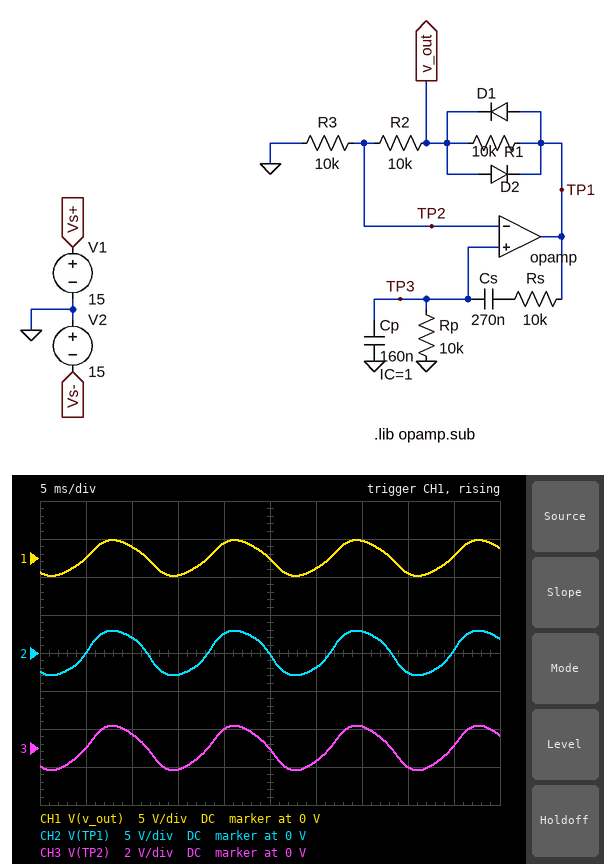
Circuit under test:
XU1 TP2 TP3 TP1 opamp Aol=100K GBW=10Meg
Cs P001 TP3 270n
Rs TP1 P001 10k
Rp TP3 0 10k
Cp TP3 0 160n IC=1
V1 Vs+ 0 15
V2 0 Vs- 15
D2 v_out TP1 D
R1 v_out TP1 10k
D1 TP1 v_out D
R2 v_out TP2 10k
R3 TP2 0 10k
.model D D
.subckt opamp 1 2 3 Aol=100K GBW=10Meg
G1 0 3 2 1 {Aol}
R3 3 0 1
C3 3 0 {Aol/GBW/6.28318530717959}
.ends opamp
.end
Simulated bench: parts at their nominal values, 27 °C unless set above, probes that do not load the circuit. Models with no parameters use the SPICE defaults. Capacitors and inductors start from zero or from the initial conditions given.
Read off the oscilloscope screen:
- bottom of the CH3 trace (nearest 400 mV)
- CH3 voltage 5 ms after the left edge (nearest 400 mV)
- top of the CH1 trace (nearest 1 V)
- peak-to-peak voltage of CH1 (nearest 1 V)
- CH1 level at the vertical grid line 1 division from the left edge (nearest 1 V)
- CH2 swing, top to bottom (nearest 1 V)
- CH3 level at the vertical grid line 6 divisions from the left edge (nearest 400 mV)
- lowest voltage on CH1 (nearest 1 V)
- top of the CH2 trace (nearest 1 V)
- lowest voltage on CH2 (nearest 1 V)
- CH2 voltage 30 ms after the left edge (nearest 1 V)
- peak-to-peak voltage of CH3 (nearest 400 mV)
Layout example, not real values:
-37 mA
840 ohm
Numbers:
-1.2 V
0 V
2 V
5 V
0 V
6 V
-800 mV
-2 V
3 V
-3 V
-2 V
2.4 V
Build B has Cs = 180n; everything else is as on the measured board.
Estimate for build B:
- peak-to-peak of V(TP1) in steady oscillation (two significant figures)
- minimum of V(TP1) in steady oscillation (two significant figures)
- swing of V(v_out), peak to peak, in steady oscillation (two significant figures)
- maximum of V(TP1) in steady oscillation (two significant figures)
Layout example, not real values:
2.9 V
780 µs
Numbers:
3.8 V
-1.9 V
2.7 V
1.9 V
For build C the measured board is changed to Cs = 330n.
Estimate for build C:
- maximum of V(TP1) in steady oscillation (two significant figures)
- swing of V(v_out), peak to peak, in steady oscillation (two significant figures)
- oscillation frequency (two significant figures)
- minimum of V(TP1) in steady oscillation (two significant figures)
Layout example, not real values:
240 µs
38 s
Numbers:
3.6 V
6.0 V
68 Hz
-3.6 V
